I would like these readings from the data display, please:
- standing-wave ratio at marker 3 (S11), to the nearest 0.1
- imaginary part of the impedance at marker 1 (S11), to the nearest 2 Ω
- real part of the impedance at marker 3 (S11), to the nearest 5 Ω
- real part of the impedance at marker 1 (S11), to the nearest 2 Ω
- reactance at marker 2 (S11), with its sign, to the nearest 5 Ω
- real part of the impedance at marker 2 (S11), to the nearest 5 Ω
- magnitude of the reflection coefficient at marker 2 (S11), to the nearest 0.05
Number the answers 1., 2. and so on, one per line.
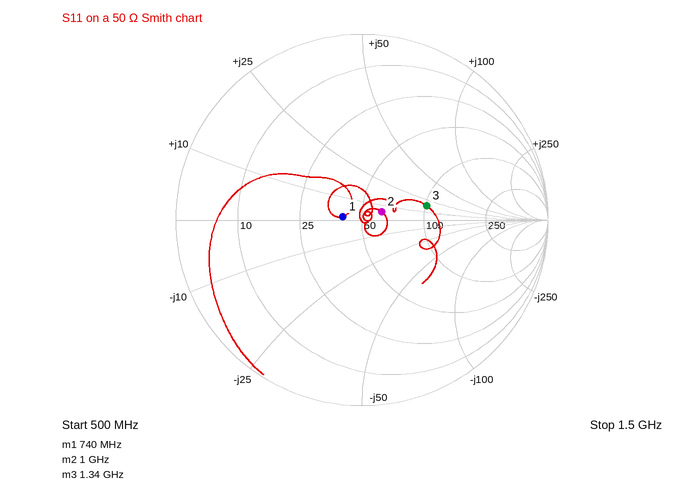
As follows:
1. 2.1
2. +2 Ω
3. 100 Ω
4. 40 Ω
5. +5 Ω
6. 60 Ω
7. 0.10
